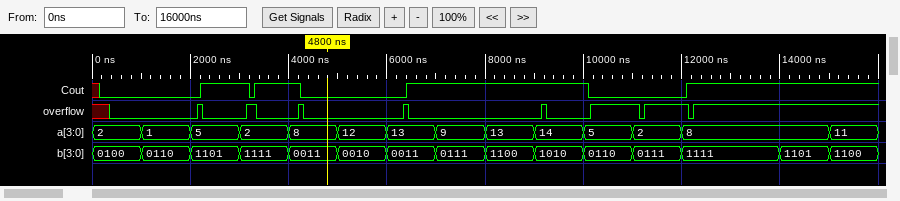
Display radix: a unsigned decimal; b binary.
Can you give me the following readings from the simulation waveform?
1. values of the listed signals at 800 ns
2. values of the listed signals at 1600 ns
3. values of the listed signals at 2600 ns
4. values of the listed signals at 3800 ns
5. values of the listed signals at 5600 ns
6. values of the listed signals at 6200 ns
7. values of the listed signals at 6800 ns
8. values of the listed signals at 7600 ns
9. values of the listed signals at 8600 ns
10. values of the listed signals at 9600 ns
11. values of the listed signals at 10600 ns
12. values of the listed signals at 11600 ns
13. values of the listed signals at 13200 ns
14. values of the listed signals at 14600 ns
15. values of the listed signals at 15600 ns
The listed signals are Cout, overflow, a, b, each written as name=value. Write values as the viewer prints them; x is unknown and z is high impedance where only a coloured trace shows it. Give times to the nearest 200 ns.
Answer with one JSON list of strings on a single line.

["Cout=0, overflow=0, a=2, b=0100", "Cout=0, overflow=0, a=1, b=0110", "Cout=1, overflow=0, a=5, b=1101", "Cout=1, overflow=0, a=2, b=1111", "Cout=0, overflow=0, a=12, b=0010", "Cout=0, overflow=0, a=13, b=0011", "Cout=1, overflow=0, a=13, b=0011", "Cout=1, overflow=0, a=9, b=0111", "Cout=1, overflow=0, a=13, b=1100", "Cout=1, overflow=0, a=14, b=1010", "Cout=0, overflow=1, a=5, b=0110", "Cout=0, overflow=1, a=2, b=0111", "Cout=1, overflow=1, a=8, b=1111", "Cout=1, overflow=1, a=8, b=1101", "Cout=1, overflow=1, a=11, b=1100"]
